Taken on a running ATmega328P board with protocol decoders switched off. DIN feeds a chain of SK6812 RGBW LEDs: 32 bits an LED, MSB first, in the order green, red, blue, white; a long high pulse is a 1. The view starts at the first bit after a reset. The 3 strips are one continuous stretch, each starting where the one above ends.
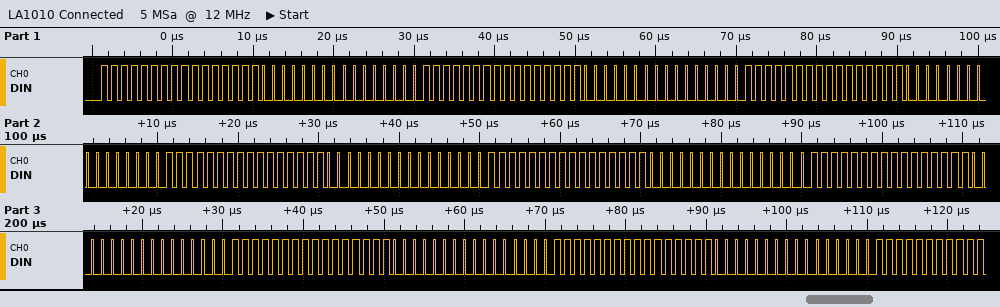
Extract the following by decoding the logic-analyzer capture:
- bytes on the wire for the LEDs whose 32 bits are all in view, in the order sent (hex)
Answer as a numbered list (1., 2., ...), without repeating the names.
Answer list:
1. FF FF 00 00 FF FF 00 00 FF FF 00 00 FF FF 00 00 FF FF 00 00 FF FF 00 00 FF FF 00 00 FF FF 00 00
